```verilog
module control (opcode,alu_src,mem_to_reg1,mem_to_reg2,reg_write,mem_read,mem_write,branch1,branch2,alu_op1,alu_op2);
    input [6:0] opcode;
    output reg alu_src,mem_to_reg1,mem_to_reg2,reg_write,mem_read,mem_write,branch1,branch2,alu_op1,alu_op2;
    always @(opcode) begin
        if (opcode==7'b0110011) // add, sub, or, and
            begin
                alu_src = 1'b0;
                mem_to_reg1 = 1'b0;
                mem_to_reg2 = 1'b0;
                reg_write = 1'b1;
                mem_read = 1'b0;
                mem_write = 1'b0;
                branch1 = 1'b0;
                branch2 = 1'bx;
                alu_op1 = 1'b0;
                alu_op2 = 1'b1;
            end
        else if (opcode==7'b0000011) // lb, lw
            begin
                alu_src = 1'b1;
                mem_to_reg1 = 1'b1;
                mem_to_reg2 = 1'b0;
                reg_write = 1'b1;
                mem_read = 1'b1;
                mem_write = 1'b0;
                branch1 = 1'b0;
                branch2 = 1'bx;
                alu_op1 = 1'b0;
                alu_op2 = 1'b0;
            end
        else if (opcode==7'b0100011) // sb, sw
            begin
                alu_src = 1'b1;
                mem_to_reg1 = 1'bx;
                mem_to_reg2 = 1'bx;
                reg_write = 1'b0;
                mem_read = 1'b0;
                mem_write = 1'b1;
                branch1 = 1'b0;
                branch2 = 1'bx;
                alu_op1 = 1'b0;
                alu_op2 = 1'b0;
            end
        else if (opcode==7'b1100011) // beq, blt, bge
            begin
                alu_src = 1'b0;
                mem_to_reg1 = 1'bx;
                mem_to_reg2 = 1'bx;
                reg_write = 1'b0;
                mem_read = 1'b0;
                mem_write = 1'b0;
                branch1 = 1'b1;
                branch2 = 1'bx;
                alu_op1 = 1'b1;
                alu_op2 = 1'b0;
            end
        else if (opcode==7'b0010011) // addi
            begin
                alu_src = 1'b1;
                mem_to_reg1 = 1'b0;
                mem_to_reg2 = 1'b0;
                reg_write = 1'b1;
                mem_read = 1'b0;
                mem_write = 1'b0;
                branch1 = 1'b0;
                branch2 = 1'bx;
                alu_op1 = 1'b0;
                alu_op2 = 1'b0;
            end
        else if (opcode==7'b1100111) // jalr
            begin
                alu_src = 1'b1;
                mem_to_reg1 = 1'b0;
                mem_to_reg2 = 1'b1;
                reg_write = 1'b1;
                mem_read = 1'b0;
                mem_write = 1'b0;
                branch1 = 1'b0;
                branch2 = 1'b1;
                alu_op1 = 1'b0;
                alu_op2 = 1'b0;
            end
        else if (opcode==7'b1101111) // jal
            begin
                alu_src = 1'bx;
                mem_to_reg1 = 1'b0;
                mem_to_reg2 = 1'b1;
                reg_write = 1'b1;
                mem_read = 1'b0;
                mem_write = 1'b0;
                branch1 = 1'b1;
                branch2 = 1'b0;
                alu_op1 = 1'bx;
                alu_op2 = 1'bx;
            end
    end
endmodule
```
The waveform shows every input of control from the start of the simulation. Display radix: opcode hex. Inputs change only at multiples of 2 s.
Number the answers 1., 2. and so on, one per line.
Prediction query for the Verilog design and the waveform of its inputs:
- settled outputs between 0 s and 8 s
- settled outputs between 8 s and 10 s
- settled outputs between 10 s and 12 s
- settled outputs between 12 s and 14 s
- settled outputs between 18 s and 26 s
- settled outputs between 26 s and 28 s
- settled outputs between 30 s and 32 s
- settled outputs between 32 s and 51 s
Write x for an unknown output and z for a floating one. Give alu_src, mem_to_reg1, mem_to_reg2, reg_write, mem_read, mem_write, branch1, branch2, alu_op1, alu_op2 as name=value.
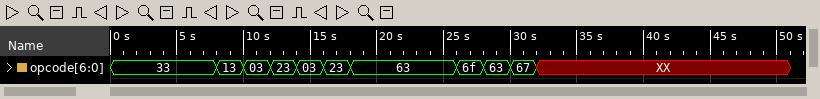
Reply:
1. alu_src=0, mem_to_reg1=0, mem_to_reg2=0, reg_write=1, mem_read=0, mem_write=0, branch1=0, branch2=x, alu_op1=0, alu_op2=1
2. alu_src=1, mem_to_reg1=0, mem_to_reg2=0, reg_write=1, mem_read=0, mem_write=0, branch1=0, branch2=x, alu_op1=0, alu_op2=0
3. alu_src=1, mem_to_reg1=1, mem_to_reg2=0, reg_write=1, mem_read=1, mem_write=0, branch1=0, branch2=x, alu_op1=0, alu_op2=0
4. alu_src=1, mem_to_reg1=x, mem_to_reg2=x, reg_write=0, mem_read=0, mem_write=1, branch1=0, branch2=x, alu_op1=0, alu_op2=0
5. alu_src=0, mem_to_reg1=x, mem_to_reg2=x, reg_write=0, mem_read=0, mem_write=0, branch1=1, branch2=x, alu_op1=1, alu_op2=0
6. alu_src=x, mem_to_reg1=0, mem_to_reg2=1, reg_write=1, mem_read=0, mem_write=0, branch1=1, branch2=0, alu_op1=x, alu_op2=x
7. alu_src=1, mem_to_reg1=0, mem_to_reg2=1, reg_write=1, mem_read=0, mem_write=0, branch1=0, branch2=1, alu_op1=0, alu_op2=0
8. alu_src=1, mem_to_reg1=0, mem_to_reg2=1, reg_write=1, mem_read=0, mem_write=0, branch1=0, branch2=1, alu_op1=0, alu_op2=0
